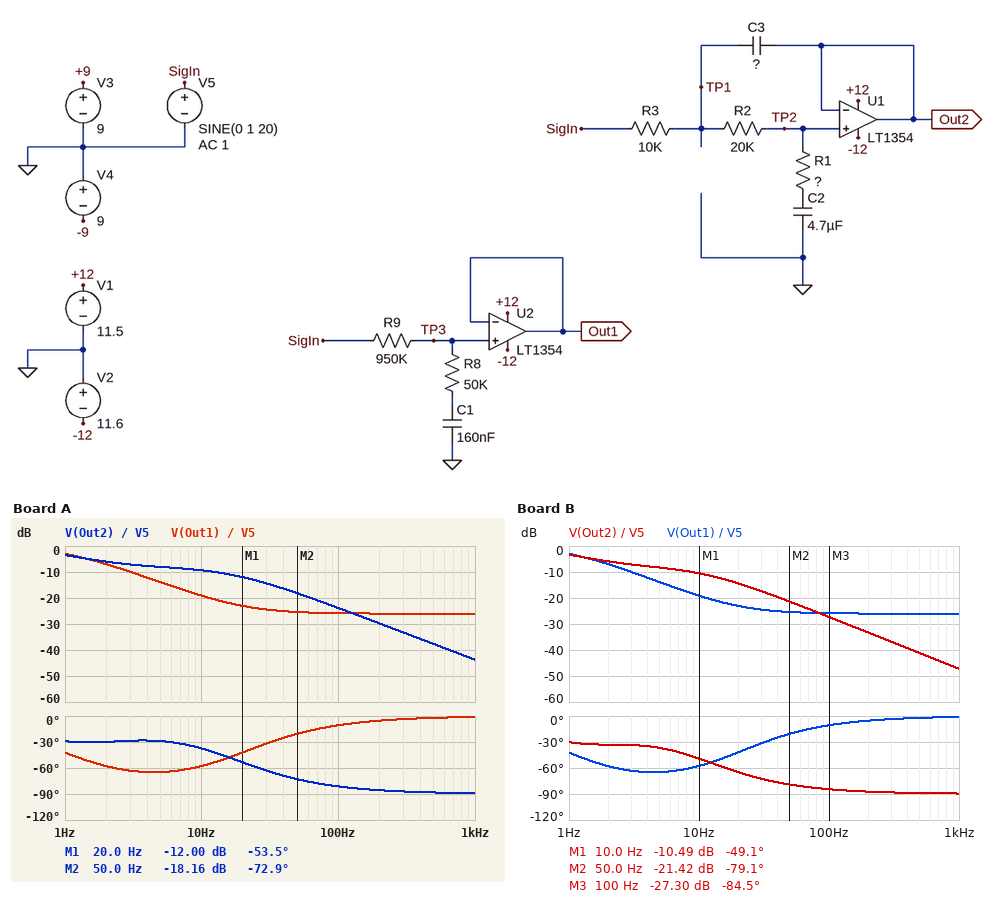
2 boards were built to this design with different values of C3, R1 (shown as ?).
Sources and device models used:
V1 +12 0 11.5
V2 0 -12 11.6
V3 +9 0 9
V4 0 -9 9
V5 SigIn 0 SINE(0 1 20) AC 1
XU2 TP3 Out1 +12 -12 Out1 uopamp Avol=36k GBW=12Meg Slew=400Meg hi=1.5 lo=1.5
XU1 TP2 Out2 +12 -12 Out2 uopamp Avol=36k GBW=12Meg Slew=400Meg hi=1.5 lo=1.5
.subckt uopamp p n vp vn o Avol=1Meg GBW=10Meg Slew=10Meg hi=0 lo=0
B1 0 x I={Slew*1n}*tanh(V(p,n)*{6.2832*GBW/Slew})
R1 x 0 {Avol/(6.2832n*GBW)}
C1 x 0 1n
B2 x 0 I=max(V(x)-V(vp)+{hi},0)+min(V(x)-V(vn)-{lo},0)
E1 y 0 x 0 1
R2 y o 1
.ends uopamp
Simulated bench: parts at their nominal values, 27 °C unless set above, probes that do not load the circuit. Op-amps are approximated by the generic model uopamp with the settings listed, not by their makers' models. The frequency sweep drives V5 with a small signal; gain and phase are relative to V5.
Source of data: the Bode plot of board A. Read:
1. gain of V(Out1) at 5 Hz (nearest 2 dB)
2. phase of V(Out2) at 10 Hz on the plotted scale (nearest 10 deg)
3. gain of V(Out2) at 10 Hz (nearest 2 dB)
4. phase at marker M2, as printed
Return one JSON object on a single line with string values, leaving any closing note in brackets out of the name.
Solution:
{"gain of V(Out1) at 5 Hz": "-14 dB", "phase of V(Out2) at 10 Hz on the plotted scale": "-40 deg", "gain of V(Out2) at 10 Hz": "-10 dB", "phase at marker M2, as printed": "-72.9 deg"}
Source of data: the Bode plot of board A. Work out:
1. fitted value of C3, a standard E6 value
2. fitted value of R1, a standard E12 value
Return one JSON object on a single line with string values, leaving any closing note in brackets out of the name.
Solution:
{"fitted value of C3, a standard E6 value": "2.2 µF", "fitted value of R1, a standard E12 value": "18 kΩ"}
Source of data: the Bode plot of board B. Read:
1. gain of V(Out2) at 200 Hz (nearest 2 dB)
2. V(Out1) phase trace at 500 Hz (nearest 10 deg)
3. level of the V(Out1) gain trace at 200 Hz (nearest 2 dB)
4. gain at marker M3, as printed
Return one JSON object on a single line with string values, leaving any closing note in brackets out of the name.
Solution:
{"gain of V(Out2) at 200 Hz": "-34 dB", "V(Out1) phase trace at 500 Hz": "0 deg", "level of the V(Out1) gain trace at 200 Hz": "-26 dB", "gain at marker M3, as printed": "-27.30 dB"}
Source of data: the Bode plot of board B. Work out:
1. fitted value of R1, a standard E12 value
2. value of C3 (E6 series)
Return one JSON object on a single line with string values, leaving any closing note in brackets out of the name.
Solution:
{"fitted value of R1, a standard E12 value": "18 kΩ", "value of C3": "3.3 µF"}
